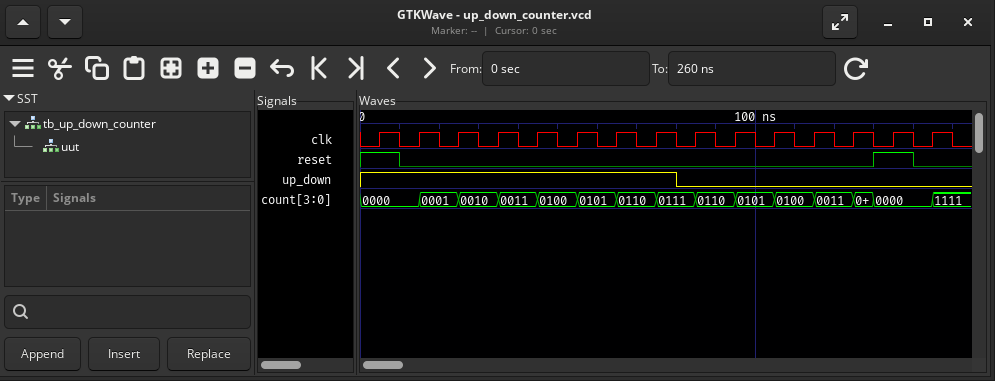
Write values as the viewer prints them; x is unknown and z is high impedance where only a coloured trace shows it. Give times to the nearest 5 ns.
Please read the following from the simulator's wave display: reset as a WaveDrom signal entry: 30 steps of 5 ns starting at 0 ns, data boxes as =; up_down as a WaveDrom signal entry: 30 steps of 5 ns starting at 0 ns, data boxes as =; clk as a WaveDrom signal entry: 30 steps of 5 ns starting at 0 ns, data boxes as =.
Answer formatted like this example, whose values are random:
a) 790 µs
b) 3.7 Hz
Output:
a) {name: 'reset', wave: '1.0.......................1.0.'}
b) {name: 'up_down', wave: '1...............0.............'}
c) {name: 'clk', wave: '010101010101010101010101010101'}
